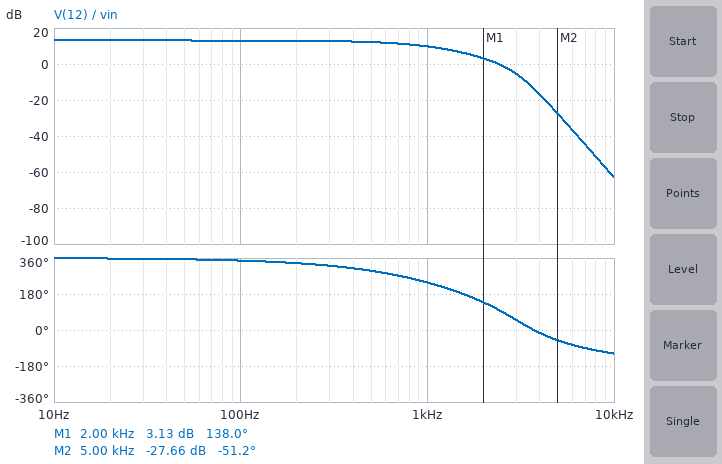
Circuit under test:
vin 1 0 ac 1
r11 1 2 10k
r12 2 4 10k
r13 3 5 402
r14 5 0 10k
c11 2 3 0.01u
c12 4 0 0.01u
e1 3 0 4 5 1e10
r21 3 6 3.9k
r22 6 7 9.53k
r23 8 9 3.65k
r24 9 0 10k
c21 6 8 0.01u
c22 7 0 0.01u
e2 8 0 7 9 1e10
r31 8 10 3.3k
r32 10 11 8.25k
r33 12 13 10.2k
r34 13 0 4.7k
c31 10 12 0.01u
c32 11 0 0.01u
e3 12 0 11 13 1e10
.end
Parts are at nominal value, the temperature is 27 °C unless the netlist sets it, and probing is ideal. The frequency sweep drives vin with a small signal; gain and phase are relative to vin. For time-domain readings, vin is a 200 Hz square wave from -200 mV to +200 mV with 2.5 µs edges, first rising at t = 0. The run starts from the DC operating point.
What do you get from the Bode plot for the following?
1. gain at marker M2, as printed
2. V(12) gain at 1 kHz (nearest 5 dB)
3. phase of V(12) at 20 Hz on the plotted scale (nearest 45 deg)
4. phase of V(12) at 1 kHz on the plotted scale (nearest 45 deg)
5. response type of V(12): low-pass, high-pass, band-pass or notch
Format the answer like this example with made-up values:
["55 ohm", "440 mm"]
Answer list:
["-27.66 dB", "10 dB", "360 deg", "225 deg", "low-pass"]
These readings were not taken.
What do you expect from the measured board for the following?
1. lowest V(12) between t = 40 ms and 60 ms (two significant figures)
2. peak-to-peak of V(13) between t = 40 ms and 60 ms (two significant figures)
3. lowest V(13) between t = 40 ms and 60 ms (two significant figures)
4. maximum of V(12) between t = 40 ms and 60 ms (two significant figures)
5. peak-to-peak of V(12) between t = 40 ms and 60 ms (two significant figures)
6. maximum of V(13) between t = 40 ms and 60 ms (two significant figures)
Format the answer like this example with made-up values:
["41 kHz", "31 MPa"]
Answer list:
["-900 mV", "570 mV", "-280 mV", "900 mV", "1.8 V", "280 mV"]
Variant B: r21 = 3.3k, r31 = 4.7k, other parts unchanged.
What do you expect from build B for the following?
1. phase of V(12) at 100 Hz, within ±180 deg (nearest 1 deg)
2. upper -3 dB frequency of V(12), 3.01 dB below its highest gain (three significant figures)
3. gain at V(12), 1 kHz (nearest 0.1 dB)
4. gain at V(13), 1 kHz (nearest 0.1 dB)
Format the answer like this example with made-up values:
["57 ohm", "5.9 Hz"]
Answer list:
["-12 deg", "1.09 kHz", "10.4 dB", "0.4 dB"]
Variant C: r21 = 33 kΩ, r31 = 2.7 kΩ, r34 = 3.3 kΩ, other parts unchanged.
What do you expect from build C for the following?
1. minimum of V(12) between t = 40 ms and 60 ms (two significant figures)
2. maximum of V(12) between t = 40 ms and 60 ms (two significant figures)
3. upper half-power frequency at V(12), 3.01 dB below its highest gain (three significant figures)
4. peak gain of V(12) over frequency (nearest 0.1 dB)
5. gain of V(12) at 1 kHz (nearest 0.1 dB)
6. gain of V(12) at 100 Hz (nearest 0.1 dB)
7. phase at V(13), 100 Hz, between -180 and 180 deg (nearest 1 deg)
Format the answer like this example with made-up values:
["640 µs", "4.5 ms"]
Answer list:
["-1.2 V", "1.2 V", "605 Hz", "15.3 dB", "7.5 dB", "15.2 dB", "-19 deg"]
